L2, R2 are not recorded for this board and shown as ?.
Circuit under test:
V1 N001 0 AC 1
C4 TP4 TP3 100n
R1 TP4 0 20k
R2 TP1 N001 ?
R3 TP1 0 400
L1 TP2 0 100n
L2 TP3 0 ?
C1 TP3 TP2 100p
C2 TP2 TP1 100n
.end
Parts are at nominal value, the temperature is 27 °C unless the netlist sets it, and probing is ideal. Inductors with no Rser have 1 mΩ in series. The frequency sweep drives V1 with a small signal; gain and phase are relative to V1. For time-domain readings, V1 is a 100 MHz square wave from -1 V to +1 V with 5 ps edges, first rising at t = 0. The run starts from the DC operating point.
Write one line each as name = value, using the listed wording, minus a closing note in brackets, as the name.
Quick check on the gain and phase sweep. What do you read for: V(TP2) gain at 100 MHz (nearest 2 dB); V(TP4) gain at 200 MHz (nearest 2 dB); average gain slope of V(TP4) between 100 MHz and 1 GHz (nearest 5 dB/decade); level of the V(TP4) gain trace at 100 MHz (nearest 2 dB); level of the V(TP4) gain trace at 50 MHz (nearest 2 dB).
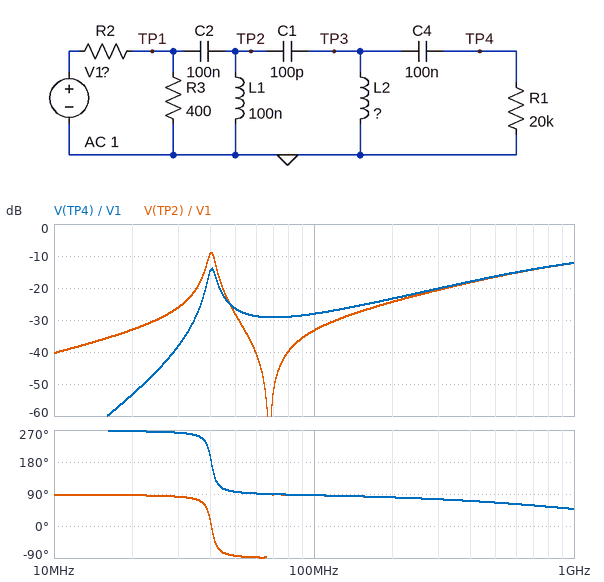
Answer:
V(TP2) gain at 100 MHz = -34 dB
V(TP4) gain at 200 MHz = -24 dB
average gain slope of V(TP4) between 100 MHz and 1 GHz = 15 dB/decade
level of the V(TP4) gain trace at 100 MHz = -28 dB
level of the V(TP4) gain trace at 50 MHz = -26 dB
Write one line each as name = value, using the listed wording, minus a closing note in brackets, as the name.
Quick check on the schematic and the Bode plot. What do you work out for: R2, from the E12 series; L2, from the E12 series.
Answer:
R2, from the E12 series = 680 Ω
L2, from the E12 series = 56 nH
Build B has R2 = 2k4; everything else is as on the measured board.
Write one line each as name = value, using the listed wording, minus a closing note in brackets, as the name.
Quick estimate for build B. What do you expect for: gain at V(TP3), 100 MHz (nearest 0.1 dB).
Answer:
gain at V(TP3), 100 MHz = -39.0 dB
